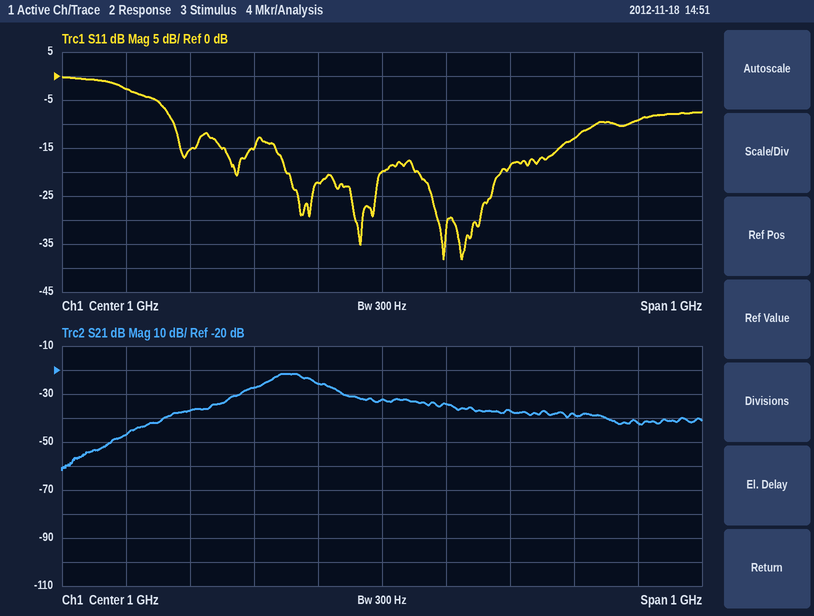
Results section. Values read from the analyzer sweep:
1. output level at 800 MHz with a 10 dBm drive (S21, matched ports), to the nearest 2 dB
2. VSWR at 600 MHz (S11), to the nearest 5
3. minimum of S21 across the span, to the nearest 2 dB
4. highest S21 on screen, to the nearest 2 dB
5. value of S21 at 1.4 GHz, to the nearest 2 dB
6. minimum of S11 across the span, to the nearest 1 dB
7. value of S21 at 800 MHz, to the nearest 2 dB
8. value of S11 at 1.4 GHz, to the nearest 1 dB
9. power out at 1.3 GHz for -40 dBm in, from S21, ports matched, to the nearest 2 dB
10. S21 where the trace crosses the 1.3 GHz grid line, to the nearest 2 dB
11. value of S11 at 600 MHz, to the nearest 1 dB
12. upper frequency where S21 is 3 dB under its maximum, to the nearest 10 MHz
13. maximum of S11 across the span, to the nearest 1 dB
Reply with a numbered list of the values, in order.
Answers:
1. -18 dBm
2. 5
3. -62 dB
4. -22 dB
5. -42 dB
6. -38 dB
7. -28 dB
8. -9 dB
9. -78 dBm
10. -38 dB
11. -3 dB
12. 890 MHz
13. 0 dB
